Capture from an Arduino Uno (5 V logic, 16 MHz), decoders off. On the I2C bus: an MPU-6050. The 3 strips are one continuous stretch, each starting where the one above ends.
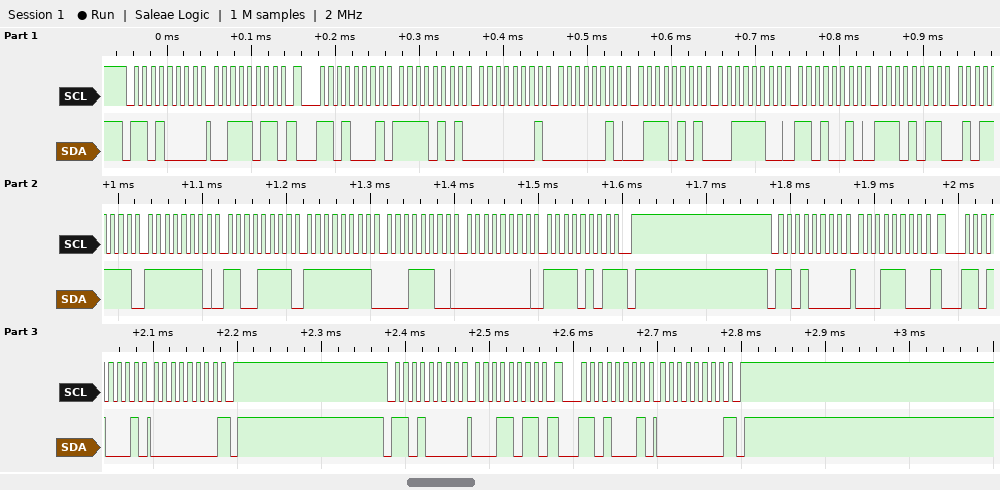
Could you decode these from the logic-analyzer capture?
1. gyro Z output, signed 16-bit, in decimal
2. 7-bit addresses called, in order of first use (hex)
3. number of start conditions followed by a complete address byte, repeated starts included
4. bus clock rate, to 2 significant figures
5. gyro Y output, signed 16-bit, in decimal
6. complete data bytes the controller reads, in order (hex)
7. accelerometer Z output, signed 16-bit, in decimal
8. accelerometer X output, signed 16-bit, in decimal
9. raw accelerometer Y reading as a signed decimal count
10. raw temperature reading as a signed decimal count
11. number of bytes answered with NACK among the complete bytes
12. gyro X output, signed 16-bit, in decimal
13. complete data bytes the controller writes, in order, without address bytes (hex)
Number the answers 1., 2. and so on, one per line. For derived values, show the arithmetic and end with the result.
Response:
1. 0x00F5 = 245
2. 0x68
3. 6
4. 100 kHz
5. 0xFF1C = -228
6. F5 01 02 75 3C D2 EB 5F FE CF FF 1C 00 F5 00 00
7. 0x3CD2 = 15570
8. 0xF501 = -2815
9. 0x0275 = 629
10. 0xEB5F = -5281
11. 3
12. 0xFECF = -305
13. 3B 1C 1B
